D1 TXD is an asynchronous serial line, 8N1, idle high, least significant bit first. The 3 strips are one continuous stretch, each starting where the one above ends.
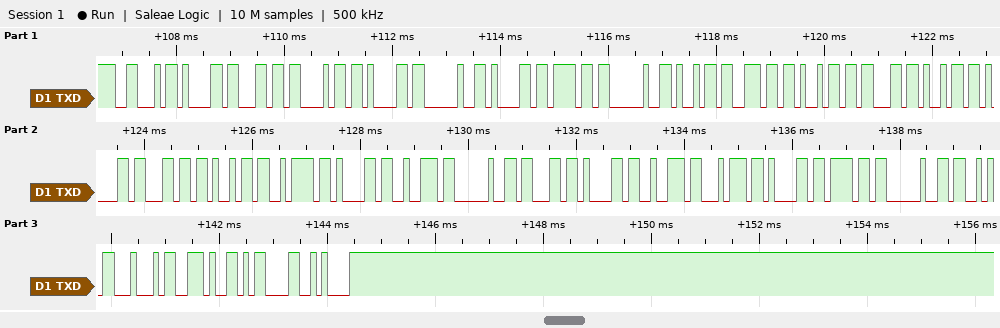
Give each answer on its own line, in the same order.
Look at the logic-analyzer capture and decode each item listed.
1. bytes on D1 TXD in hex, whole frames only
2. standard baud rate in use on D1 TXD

0x46 0x61 0x6C 0x68 0x61 0x20 0x61 0x6F 0x20 0x69 0x6E 0x69 0x63 0x69 0x61 0x6C 0x69 0x7A 0x61 0x72 0x20 0x63 0x61 0x72 0x74 0x61 0x6F 0x20 0x53 0x44 0x2E 0x0D 0x0A
9600 baud
